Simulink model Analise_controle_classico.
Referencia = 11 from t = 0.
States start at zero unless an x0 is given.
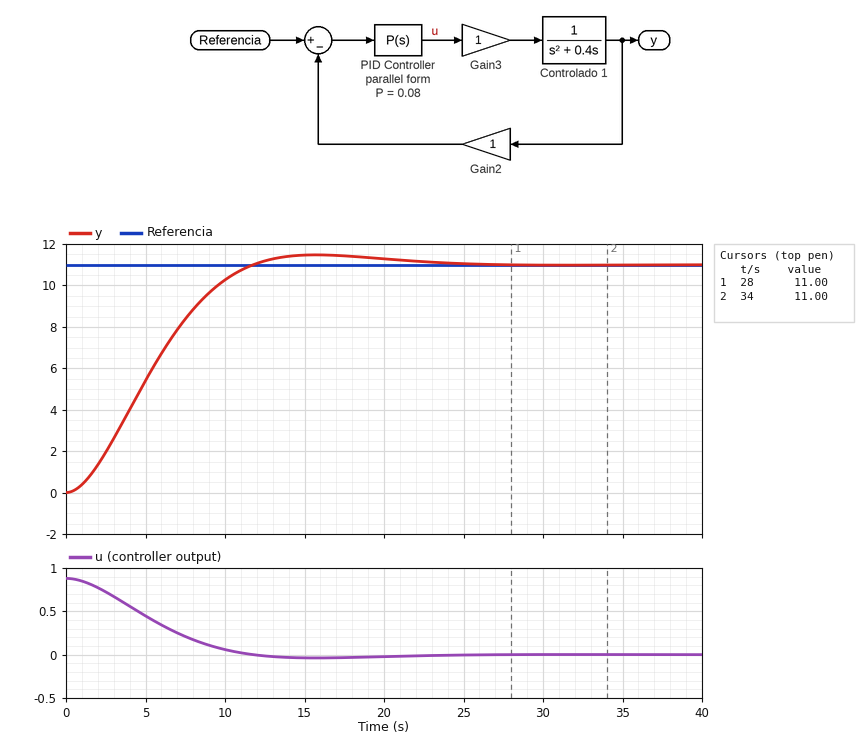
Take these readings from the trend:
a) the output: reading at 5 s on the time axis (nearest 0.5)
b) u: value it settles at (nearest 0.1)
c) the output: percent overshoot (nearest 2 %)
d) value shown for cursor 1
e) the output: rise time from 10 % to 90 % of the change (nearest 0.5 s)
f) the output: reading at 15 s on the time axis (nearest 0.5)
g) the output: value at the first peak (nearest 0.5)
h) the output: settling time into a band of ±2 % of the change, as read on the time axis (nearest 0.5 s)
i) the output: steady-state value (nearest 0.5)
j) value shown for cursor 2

5.5
0.0
4 %
11.00
7.5 s
11.5
11.5
21.0 s
11.0
11.00
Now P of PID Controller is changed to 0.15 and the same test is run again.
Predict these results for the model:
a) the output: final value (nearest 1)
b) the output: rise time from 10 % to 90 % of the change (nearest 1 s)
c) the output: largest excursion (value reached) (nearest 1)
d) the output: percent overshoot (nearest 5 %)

11
4 s
13
15 %
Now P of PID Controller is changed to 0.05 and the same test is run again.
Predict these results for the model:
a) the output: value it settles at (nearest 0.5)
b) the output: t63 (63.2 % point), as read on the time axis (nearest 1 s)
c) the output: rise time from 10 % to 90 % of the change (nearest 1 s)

11.0
9 s
13 s
